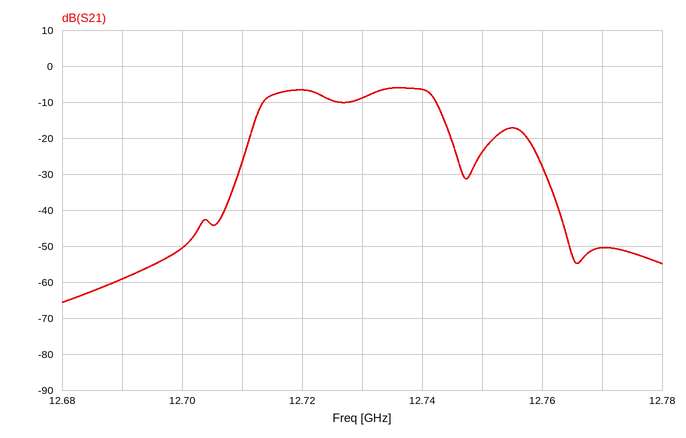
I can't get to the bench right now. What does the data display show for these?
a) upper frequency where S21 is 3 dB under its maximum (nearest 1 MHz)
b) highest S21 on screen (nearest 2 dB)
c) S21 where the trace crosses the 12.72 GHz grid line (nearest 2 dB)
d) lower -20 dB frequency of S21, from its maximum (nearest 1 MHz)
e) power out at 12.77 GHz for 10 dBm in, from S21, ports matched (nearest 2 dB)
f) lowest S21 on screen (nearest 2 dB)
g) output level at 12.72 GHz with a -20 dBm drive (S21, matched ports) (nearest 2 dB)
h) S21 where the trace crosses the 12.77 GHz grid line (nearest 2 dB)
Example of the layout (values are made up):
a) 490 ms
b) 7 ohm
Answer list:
a) 12.742 GHz
b) -6 dB
c) -6 dB
d) 12.710 GHz
e) -40 dBm
f) -66 dB
g) -26 dBm
h) -50 dB
